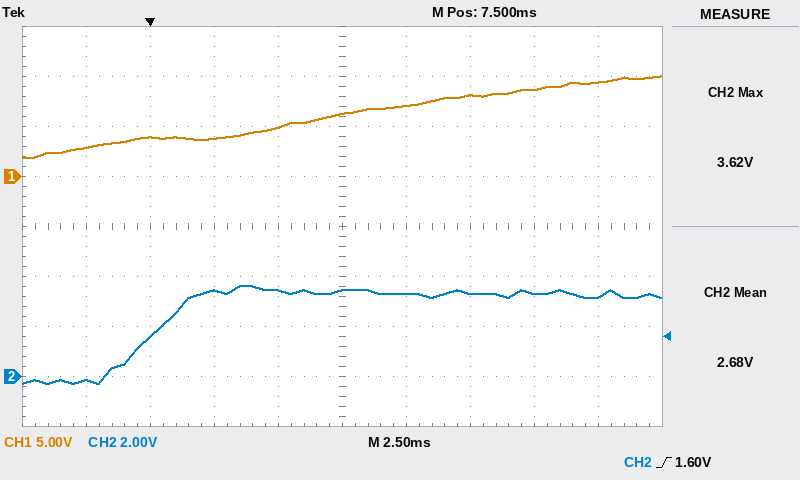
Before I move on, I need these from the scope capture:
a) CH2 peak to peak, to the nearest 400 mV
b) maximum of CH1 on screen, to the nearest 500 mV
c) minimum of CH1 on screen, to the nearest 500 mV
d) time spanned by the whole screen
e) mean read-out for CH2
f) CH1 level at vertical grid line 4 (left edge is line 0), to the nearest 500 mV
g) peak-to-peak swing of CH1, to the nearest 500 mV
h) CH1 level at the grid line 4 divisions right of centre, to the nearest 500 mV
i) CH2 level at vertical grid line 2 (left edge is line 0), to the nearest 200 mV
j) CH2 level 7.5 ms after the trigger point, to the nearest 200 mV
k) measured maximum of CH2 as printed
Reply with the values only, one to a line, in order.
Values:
4.0 V
10.0 V
2.0 V
25 ms
2.68 V
5.0 V
8.0 V
9.5 V
1.6 V
3.4 V
3.62 V
